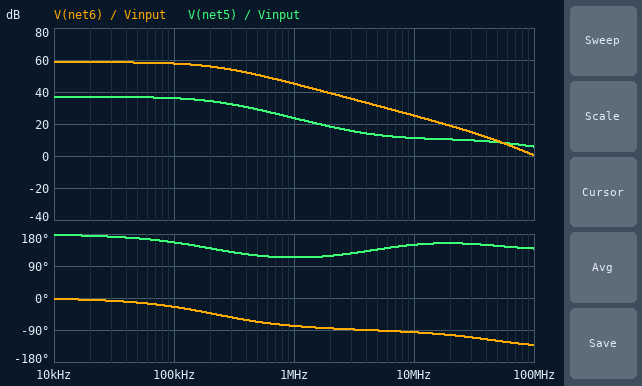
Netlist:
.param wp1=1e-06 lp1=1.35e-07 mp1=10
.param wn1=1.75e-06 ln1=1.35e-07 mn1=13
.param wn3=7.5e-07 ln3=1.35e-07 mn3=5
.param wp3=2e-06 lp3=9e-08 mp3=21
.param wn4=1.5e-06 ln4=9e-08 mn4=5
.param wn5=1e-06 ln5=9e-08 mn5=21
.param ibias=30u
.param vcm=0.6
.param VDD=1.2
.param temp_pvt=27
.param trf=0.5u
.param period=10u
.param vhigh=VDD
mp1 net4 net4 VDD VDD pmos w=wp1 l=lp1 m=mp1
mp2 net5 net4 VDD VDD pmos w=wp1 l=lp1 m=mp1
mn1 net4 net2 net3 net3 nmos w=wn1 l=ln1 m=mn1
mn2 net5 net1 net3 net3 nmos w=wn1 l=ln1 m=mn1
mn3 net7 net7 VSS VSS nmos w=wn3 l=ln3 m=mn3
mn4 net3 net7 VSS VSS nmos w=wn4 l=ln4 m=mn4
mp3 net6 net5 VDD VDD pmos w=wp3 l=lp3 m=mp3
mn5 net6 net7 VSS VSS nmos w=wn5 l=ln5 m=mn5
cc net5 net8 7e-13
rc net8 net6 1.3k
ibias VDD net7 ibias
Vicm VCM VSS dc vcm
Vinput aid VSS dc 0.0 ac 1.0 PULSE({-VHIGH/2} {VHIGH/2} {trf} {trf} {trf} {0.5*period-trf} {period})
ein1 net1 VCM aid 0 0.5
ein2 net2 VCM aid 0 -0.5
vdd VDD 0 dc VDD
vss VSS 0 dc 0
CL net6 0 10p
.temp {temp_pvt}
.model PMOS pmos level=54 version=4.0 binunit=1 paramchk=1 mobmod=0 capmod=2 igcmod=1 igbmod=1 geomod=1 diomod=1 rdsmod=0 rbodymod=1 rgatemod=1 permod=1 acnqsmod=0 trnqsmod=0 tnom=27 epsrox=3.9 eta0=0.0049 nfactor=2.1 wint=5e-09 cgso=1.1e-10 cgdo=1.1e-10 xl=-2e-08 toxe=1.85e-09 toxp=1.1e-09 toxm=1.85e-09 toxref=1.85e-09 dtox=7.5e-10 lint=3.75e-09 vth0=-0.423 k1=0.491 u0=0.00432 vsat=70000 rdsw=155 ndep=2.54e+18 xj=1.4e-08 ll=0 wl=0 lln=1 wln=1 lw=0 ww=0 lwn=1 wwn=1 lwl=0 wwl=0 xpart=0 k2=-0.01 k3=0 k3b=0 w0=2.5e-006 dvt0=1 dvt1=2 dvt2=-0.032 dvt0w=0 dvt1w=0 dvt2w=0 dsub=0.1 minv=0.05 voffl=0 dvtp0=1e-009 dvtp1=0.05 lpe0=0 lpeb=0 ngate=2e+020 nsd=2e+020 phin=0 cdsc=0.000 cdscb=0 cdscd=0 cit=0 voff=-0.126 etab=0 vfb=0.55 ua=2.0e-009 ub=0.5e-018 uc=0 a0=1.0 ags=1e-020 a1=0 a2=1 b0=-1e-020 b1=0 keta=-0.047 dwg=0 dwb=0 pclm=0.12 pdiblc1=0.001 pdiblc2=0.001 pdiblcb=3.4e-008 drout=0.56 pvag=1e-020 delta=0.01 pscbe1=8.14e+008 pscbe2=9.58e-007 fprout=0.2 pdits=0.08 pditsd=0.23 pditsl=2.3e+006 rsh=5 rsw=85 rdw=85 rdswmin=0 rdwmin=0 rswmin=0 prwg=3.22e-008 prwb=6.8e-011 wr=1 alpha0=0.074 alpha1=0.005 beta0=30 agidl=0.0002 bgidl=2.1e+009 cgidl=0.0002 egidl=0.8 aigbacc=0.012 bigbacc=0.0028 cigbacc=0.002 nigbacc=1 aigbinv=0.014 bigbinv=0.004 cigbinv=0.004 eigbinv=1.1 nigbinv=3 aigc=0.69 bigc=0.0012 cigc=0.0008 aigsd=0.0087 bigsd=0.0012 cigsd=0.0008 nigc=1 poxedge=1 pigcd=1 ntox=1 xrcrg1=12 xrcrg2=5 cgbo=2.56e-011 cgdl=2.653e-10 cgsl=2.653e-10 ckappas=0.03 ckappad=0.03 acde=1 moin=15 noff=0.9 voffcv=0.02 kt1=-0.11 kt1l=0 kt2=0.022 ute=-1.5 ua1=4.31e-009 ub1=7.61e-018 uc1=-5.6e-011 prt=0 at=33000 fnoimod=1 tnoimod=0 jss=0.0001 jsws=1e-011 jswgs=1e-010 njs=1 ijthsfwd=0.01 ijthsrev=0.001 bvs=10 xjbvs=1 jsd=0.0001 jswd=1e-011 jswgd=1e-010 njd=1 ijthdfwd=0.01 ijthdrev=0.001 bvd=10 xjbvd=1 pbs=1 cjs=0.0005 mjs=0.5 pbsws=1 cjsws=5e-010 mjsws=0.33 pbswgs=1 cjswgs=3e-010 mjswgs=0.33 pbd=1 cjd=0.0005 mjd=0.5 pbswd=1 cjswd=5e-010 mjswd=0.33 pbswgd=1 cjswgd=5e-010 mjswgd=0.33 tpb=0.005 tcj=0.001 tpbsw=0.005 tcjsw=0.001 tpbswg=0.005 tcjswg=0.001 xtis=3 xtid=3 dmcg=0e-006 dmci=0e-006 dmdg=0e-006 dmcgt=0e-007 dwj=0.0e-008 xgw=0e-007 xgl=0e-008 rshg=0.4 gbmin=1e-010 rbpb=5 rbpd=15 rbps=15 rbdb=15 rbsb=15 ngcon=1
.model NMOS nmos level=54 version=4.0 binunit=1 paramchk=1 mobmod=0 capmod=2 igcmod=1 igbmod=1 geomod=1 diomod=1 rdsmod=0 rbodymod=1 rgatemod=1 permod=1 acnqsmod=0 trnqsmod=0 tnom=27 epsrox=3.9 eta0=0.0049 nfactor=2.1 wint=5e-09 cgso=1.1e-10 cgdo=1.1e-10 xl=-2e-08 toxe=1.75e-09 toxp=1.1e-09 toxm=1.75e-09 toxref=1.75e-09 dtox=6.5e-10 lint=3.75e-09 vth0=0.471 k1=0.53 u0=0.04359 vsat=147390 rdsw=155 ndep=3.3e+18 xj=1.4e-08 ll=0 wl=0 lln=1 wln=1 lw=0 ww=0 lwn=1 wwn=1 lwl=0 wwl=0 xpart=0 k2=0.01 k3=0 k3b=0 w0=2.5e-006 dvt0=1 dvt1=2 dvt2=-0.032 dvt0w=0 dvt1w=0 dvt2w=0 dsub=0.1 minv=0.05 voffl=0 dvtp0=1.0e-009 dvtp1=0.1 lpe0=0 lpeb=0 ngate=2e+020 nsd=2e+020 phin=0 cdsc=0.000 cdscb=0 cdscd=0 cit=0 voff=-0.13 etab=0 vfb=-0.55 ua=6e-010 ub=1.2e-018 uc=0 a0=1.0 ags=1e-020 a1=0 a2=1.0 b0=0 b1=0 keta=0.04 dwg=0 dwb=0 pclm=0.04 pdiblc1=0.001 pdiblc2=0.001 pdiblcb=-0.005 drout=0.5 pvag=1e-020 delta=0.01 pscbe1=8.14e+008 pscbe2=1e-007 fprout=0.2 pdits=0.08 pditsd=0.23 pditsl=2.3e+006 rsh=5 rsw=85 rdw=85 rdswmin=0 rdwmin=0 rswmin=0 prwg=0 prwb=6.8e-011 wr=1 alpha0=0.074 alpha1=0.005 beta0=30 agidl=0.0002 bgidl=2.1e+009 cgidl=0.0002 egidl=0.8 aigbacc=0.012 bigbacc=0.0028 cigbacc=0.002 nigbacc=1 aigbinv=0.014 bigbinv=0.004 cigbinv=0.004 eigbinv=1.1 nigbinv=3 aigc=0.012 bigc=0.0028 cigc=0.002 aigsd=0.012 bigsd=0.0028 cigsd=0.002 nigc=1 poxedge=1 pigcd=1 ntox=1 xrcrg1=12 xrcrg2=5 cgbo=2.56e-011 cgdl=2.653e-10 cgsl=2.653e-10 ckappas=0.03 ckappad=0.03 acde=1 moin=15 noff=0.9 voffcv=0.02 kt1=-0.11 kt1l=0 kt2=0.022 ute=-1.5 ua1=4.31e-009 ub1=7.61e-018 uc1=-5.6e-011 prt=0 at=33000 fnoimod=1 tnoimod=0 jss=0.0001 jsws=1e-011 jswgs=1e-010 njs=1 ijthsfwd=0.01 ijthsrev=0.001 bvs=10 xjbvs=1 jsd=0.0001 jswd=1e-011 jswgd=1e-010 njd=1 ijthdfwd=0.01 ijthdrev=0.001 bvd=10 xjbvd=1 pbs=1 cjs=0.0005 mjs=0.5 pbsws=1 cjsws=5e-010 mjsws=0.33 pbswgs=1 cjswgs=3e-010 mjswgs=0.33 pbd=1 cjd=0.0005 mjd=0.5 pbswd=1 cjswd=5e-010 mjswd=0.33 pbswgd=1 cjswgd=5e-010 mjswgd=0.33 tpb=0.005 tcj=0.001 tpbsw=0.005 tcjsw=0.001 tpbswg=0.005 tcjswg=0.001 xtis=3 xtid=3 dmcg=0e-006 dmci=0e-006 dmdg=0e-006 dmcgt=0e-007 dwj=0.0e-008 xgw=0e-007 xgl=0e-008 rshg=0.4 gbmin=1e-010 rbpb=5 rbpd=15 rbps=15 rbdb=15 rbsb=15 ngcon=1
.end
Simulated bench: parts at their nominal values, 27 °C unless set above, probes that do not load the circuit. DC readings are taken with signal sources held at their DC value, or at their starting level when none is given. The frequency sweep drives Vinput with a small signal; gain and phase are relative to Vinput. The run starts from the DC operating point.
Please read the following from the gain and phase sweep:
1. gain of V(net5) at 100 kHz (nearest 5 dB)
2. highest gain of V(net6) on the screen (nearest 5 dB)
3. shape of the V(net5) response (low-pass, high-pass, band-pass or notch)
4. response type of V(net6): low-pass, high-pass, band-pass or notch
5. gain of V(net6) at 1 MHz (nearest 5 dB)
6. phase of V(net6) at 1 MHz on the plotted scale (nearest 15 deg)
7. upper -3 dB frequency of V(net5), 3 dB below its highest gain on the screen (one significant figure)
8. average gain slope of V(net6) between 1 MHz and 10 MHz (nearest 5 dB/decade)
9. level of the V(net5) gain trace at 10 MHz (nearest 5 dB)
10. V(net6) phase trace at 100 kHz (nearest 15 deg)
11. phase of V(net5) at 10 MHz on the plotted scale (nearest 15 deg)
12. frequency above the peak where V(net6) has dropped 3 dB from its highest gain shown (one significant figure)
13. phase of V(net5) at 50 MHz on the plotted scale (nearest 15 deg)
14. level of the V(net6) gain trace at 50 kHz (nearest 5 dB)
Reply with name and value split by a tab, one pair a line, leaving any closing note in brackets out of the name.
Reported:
gain of V(net5) at 100 kHz	35 dB
highest gain of V(net6) on the screen	60 dB
shape of the V(net5) response	low-pass
response type of V(net6): low-pass, high-pass, band-pass or notch	low-pass
gain of V(net6) at 1 MHz	45 dB
phase of V(net6) at 1 MHz on the plotted scale	-75 deg
upper -3 dB frequency of V(net5), 3 dB below its highest gain on the screen	200 kHz
average gain slope of V(net6) between 1 MHz and 10 MHz	-20 dB/decade
level of the V(net5) gain trace at 10 MHz	10 dB
V(net6) phase trace at 100 kHz	-30 deg
phase of V(net5) at 10 MHz on the plotted scale	150 deg
frequency above the peak where V(net6) has dropped 3 dB from its highest gain shown	200 kHz
phase of V(net5) at 50 MHz on the plotted scale	150 deg
level of the V(net6) gain trace at 50 kHz	60 dB
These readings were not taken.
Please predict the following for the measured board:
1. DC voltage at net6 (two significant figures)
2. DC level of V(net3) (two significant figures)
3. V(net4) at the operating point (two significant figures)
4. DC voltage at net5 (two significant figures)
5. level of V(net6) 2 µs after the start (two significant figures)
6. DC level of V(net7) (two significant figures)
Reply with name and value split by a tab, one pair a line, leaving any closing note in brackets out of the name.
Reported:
DC voltage at net6	980 mV
DC level of V(net3)	200 mV
V(net4) at the operating point	640 mV
DC voltage at net5	640 mV
level of V(net6) 2 µs after the start	1.2 V
DC level of V(net7)	470 mV
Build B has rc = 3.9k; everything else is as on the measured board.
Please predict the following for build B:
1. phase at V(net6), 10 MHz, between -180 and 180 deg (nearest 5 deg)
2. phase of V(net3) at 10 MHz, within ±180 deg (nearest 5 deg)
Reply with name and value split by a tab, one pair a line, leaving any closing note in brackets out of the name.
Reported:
phase at V(net6), 10 MHz, between -180 and 180 deg	-90 deg
phase of V(net3) at 10 MHz, within ±180 deg	165 deg
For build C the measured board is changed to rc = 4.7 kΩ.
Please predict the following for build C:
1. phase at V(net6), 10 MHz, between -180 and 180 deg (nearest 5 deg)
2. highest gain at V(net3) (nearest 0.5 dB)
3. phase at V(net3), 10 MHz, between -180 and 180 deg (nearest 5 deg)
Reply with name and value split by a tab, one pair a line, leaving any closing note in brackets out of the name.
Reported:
phase at V(net6), 10 MHz, between -180 and 180 deg	-90 deg
highest gain at V(net3)	-10.5 dB
phase at V(net3), 10 MHz, between -180 and 180 deg	165 deg
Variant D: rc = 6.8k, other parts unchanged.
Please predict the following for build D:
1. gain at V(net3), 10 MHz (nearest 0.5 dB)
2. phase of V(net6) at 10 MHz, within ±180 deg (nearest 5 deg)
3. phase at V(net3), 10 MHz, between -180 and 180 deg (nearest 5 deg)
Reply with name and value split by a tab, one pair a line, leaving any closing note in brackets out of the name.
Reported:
gain at V(net3), 10 MHz	-33.0 dB
phase of V(net6) at 10 MHz, within ±180 deg	-85 deg
phase at V(net3), 10 MHz, between -180 and 180 deg	170 deg
